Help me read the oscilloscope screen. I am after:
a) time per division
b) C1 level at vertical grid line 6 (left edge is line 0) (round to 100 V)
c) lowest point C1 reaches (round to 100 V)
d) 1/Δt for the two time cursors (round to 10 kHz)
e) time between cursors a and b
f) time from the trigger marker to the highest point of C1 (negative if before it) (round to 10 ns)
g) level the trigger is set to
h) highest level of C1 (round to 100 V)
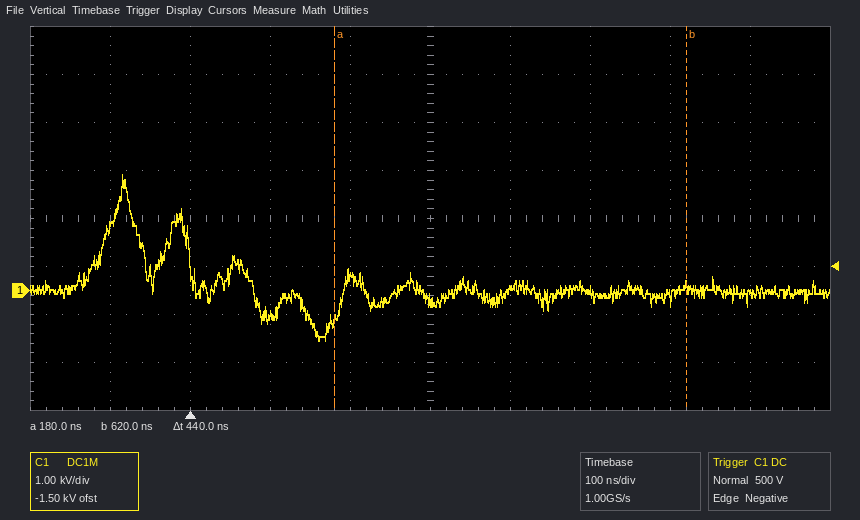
100 ns
0.0 kV
-1.0 kV
2.27 MHz
440 ns
-80 ns
500 V
2.4 kV
